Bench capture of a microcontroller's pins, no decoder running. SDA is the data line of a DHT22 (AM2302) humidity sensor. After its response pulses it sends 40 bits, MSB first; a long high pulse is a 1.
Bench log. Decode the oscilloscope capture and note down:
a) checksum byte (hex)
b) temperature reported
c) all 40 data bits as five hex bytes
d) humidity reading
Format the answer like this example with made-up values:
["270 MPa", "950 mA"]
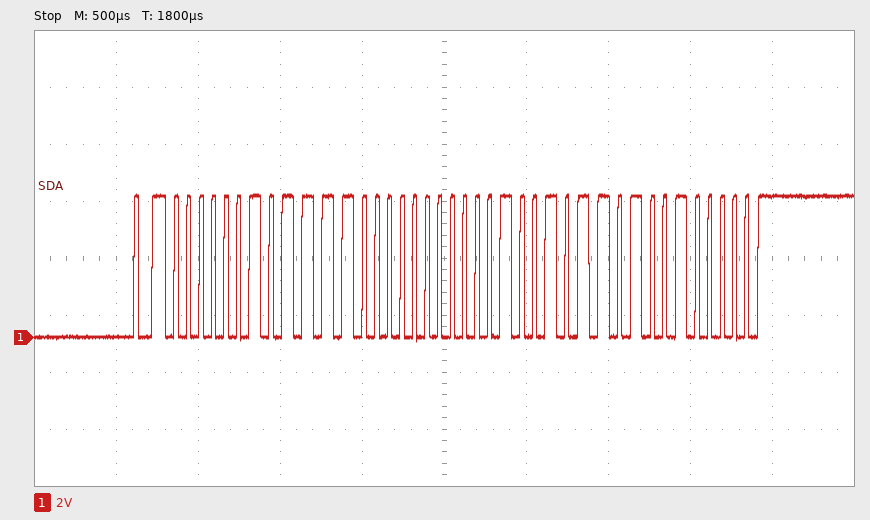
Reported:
["0x20", "30.1 °C", "02 F0 01 2D 20", "75.2 %"]
